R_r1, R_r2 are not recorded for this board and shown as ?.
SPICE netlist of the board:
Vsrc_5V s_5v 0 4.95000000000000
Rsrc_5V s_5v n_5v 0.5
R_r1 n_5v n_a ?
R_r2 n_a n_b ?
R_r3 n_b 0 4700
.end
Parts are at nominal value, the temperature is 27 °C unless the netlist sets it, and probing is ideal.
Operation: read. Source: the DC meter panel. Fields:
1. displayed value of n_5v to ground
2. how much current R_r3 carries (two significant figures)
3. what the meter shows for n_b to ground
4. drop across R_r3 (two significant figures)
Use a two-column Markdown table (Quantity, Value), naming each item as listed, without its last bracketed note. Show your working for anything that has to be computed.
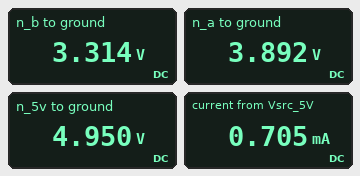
| Quantity | Value |
|---|---|
| displayed value of n_5v to ground | 4.950 V |
| how much current R_r3 carries | (3.314 V) / 4.7 kΩ = 710 µA |
| what the meter shows for n_b to ground | 3.314 V |
| drop across R_r3 | 3.314 V = 3.3 V |
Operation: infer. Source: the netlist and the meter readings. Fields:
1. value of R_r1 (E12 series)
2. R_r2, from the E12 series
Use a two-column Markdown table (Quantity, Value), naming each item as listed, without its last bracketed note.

| Quantity | Value |
|---|---|
| value of R_r1 | 1.5 kΩ |
| R_r2, from the E12 series | 820 Ω |
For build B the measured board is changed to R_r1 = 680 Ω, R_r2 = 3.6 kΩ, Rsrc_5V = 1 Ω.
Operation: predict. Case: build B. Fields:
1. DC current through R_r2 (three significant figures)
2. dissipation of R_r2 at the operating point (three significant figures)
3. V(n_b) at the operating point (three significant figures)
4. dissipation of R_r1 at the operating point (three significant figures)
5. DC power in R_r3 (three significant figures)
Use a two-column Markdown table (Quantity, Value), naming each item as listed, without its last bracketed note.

| Quantity | Value |
|---|---|
| DC current through R_r2 | 551 µA |
| dissipation of R_r2 at the operating point | 1.09 mW |
| V(n_b) at the operating point | 2.59 V |
| dissipation of R_r1 at the operating point | 207 µW |
| DC power in R_r3 | 1.43 mW |
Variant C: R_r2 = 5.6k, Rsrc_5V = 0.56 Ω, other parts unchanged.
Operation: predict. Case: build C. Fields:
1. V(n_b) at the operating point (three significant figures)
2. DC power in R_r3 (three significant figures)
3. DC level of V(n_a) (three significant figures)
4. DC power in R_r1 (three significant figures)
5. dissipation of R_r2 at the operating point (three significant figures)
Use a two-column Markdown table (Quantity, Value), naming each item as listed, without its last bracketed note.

| Quantity | Value |
|---|---|
| V(n_b) at the operating point | 1.97 V |
| DC power in R_r3 | 827 µW |
| DC level of V(n_a) | 4.32 V |
| DC power in R_r1 | 264 µW |
| dissipation of R_r2 at the operating point | 985 µW |
